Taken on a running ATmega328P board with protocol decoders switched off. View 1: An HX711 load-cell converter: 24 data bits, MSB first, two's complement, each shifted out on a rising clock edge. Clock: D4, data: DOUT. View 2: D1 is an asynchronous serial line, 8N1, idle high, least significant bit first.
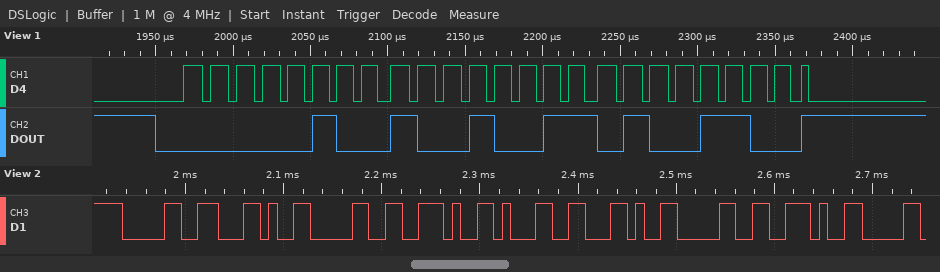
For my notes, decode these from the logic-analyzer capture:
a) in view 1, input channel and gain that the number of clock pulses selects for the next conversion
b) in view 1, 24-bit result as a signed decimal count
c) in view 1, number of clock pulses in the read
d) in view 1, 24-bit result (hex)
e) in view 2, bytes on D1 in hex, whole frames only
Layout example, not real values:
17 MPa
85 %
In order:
channel A, gain 128
299852
25
0x04934C
30 2C 30 2E 31 2C 30 2E
